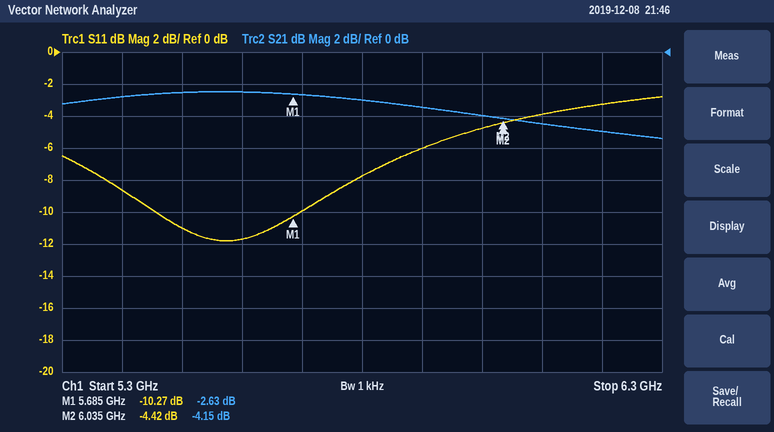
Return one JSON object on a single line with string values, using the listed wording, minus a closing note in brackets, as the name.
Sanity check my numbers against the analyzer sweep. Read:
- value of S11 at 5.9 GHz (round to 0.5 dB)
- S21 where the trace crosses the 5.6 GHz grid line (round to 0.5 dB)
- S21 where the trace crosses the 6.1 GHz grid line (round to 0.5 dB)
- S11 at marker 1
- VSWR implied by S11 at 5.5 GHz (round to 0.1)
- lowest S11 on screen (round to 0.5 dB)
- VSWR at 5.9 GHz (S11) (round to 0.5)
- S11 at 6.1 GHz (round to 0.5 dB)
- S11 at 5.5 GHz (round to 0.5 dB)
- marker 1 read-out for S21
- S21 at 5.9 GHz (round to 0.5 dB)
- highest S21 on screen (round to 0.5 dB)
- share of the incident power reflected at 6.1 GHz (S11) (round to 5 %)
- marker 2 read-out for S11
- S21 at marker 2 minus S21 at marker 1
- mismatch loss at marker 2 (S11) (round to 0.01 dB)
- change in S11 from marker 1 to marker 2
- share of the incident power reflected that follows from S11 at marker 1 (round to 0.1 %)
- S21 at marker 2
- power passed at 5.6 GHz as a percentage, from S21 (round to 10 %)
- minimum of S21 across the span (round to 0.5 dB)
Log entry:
{"value of S11 at 5.9 GHz": "-6.0 dB", "S21 where the trace crosses the 5.6 GHz grid line": "-2.5 dB", "S21 where the trace crosses the 6.1 GHz grid line": "-4.5 dB", "S11 at marker 1": "-10.27 dB", "VSWR implied by S11 at 5.5 GHz": "1.8", "lowest S11 on screen": "-12.0 dB", "VSWR at 5.9 GHz (S11)": "3.0", "S11 at 6.1 GHz": "-4.0 dB", "S11 at 5.5 GHz": "-11.0 dB", "marker 1 read-out for S21": "-2.63 dB", "S21 at 5.9 GHz": "-3.5 dB", "highest S21 on screen": "-2.5 dB", "share of the incident power reflected at 6.1 GHz (S11)": "40 %", "marker 2 read-out for S11": "-4.42 dB", "S21 at marker 2 minus S21 at marker 1": "-1.52 dB", "mismatch loss at marker 2 (S11)": "1.95 dB", "change in S11 from marker 1 to marker 2": "5.85 dB", "share of the incident power reflected that follows from S11 at marker 1": "9.4 %", "S21 at marker 2": "-4.15 dB", "power passed at 5.6 GHz as a percentage, from S21": "60 %", "minimum of S21 across the span": "-5.5 dB"}
